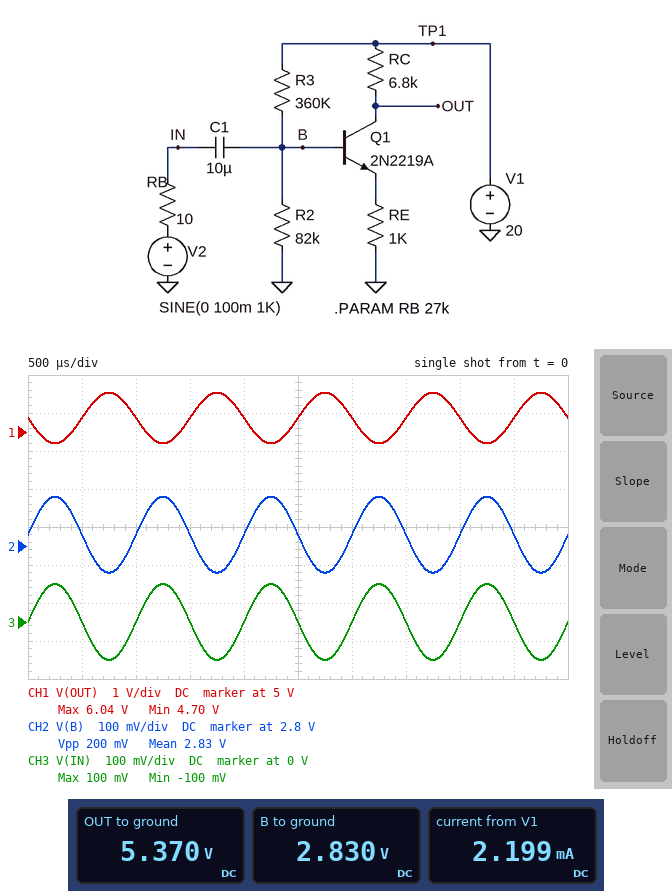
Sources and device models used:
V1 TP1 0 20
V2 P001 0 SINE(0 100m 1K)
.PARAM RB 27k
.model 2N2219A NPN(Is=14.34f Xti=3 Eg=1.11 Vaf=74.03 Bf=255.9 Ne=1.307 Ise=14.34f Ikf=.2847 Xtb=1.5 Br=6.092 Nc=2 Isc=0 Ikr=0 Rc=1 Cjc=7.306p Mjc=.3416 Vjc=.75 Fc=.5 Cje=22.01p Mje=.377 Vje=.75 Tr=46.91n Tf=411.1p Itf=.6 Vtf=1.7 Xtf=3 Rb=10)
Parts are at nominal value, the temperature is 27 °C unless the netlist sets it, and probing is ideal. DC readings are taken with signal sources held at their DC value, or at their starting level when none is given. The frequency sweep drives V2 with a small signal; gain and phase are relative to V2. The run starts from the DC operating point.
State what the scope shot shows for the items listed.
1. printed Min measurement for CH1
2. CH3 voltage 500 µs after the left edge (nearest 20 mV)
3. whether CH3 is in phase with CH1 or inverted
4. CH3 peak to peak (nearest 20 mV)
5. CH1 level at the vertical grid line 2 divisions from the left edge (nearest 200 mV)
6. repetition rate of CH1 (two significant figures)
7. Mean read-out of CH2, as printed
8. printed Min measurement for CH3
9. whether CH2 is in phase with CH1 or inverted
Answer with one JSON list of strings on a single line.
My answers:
["4.70 V", "0 V", "inverted", "200 mV", "5.4 V", "1.0 kHz", "2.83 V", "-100 mV", "inverted"]
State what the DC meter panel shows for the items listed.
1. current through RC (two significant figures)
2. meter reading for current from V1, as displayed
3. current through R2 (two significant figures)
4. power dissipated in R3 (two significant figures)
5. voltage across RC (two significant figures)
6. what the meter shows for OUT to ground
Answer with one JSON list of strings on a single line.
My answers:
["2.2 mA", "2.199 mA", "35 µA", "820 µW", "15 V", "5.370 V"]
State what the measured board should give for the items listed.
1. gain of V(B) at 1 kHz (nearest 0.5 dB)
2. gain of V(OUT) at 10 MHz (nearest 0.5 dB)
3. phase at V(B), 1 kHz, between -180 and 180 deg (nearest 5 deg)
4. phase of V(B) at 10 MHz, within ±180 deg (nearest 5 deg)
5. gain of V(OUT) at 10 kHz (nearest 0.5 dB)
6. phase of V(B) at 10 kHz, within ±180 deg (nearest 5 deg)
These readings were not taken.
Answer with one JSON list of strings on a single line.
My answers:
["0 dB", "10.0 dB", "0 deg", "0 deg", "16.5 dB", "0 deg"]
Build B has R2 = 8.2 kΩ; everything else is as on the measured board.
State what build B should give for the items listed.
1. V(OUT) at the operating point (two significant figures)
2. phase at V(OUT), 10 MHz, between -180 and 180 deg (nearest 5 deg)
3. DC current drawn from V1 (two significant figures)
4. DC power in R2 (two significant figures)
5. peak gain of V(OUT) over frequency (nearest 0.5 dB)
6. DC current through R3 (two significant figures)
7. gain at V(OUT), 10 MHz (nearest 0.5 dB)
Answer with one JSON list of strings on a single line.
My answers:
["20 V", "45 deg", "55 µA", "24 µW", "0 dB", "54 µA", "-2.5 dB"]
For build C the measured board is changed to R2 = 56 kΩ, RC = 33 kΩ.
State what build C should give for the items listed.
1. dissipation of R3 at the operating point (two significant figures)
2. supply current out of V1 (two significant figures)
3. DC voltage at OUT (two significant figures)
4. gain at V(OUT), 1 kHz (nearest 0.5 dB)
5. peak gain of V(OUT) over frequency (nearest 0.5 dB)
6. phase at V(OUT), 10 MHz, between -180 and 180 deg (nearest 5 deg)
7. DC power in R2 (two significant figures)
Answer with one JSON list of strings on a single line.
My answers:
["980 µW", "640 µA", "660 mV", "-15.5 dB", "0 dB", "5 deg", "28 µW"]
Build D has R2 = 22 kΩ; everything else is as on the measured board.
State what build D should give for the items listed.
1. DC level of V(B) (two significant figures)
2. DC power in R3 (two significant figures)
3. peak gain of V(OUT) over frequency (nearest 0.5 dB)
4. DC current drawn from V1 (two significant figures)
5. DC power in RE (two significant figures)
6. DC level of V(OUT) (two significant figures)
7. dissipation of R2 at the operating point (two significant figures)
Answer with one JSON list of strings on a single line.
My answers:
["1.1 V", "990 µW", "16.0 dB", "520 µA", "220 µW", "17 V", "54 µW"]
